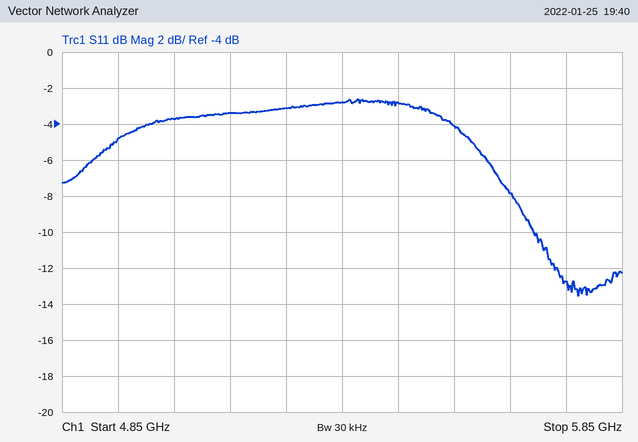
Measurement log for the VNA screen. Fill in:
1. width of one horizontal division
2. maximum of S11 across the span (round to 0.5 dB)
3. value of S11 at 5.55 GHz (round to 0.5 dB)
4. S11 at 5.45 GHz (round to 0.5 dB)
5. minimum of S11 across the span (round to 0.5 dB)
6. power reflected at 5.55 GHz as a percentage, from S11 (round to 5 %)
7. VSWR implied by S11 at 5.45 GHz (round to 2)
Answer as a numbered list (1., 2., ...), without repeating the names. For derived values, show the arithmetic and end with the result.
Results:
1. 100 MHz
2. -2.5 dB
3. -4.0 dB
4. -3.0 dB
5. -13.5 dB
6. 10^(-4/10) ≈ 40 %
7. |Γ| = 10^(-3/20) = 0.7079; VSWR = (1 + 0.7079)/(1 − 0.7079) ≈ 6
